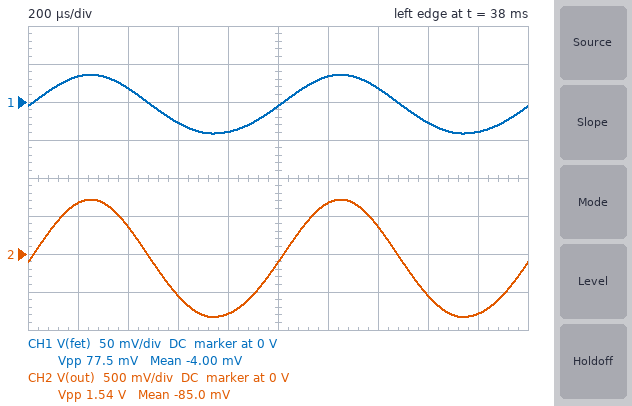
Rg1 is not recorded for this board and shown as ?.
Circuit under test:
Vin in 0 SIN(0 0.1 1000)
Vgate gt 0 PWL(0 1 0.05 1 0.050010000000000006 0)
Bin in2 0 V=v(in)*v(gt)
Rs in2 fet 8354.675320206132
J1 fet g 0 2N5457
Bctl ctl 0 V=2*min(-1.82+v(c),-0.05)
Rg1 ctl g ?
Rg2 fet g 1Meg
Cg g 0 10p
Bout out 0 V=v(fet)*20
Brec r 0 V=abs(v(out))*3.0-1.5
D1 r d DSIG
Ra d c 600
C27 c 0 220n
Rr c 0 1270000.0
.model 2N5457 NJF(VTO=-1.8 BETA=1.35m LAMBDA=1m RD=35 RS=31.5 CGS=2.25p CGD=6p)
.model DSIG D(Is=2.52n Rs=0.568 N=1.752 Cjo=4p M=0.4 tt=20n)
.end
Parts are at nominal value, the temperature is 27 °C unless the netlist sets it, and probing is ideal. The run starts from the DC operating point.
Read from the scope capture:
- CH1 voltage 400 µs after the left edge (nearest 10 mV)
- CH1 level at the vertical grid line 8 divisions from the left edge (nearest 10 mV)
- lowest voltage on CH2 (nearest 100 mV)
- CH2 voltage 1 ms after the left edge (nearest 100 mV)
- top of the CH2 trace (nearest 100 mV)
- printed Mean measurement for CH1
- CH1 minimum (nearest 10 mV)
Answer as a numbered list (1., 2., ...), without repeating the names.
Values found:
1. 20 mV
2. -30 mV
3. -800 mV
4. -100 mV
5. 700 mV
6. -4.00 mV
7. -40 mV
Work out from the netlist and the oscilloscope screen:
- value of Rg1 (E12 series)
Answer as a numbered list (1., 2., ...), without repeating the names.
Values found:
1. 390 kΩ
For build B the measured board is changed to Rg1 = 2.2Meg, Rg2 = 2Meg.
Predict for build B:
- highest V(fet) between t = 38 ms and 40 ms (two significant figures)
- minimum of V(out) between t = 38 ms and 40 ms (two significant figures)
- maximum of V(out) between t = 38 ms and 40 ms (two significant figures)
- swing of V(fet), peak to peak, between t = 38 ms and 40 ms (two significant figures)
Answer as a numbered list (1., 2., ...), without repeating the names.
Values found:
1. 26 mV
2. -600 mV
3. 520 mV
4. 56 mV
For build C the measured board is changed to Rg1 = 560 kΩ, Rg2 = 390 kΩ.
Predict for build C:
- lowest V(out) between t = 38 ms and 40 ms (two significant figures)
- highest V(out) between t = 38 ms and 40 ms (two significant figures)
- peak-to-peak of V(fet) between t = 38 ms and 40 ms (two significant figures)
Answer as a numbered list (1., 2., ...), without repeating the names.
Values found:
1. -350 mV
2. 180 mV
3. 27 mV
